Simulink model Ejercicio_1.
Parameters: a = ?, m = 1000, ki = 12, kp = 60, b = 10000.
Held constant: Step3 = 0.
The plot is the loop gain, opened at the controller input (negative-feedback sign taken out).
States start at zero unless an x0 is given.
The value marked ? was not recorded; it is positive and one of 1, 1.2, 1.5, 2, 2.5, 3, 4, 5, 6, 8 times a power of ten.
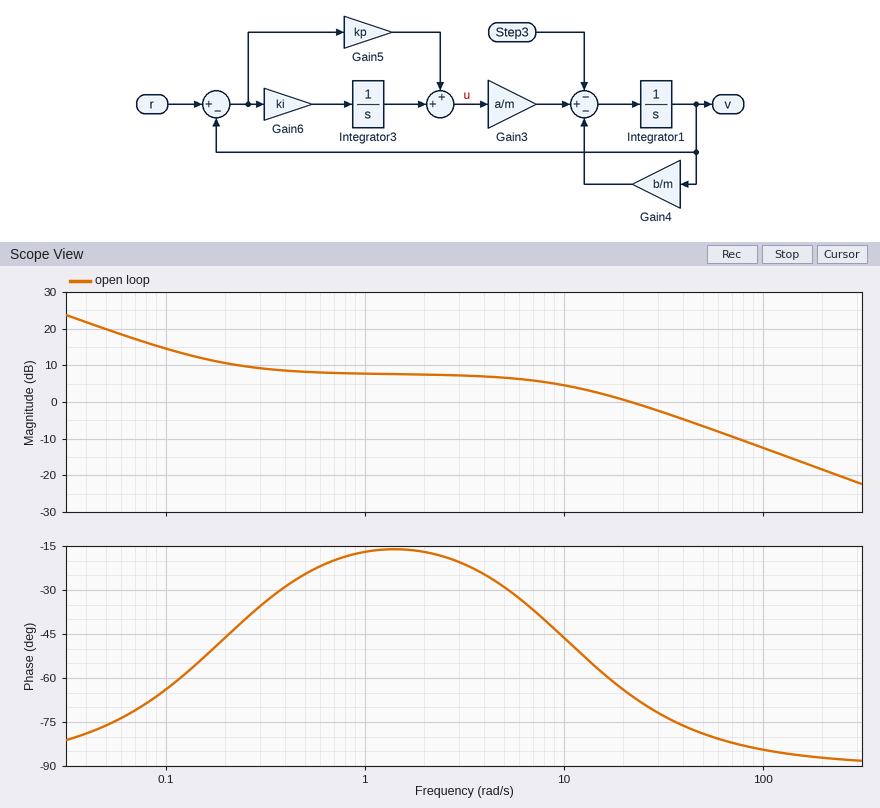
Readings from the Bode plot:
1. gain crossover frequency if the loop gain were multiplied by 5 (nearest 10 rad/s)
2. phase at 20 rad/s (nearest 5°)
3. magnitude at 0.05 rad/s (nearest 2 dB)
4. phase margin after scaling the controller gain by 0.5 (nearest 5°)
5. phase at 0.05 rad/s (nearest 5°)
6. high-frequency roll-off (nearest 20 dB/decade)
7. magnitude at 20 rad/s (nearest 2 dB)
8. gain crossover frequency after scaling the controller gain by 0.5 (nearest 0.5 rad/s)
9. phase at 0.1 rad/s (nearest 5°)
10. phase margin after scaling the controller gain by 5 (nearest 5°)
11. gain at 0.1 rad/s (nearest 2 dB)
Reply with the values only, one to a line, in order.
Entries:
120 rad/s
-65°
20 dB
145°
-75°
-20 dB/decade
0 dB
6.5 rad/s
-65°
95°
14 dB
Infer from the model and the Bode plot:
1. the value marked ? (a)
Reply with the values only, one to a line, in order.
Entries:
400
